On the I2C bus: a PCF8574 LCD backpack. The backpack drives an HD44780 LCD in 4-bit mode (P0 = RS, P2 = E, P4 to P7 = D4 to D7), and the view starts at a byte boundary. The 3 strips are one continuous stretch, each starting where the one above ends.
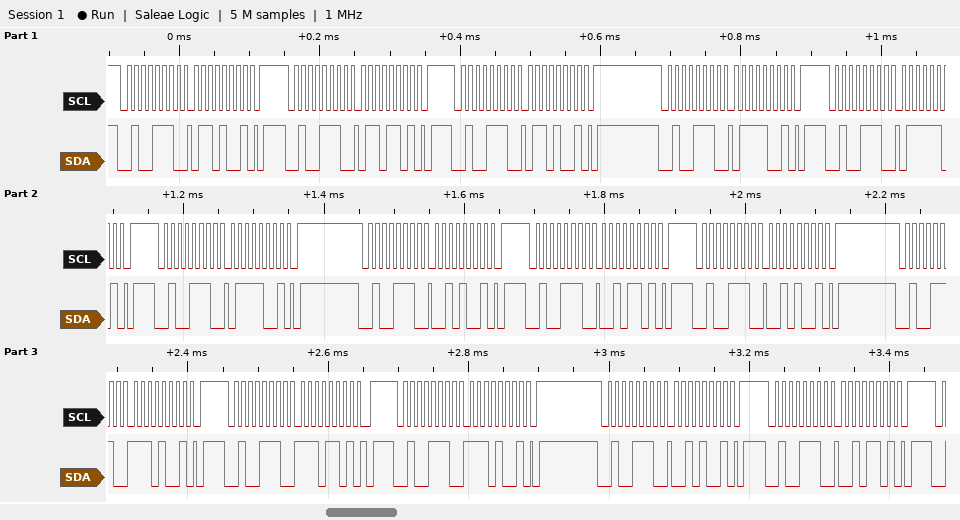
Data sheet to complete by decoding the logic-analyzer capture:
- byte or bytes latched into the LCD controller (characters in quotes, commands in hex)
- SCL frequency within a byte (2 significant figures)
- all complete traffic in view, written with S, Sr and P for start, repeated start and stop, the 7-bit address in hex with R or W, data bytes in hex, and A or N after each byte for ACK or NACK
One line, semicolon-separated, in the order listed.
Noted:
'g' '.'; 100 kHz; S 27W A 69 A P S 27W A 6D A P S 27W A 69 A P S 27W A 79 A P S 27W A 7D A P S 27W A 79 A P S 27W A 29 A P S 27W A 2D A P S 27W A 29 A P S 27W A E9 A P S 27W A ED A P S 27W A E9 A P S 27W A 29 A P S 27W A 2D A P
